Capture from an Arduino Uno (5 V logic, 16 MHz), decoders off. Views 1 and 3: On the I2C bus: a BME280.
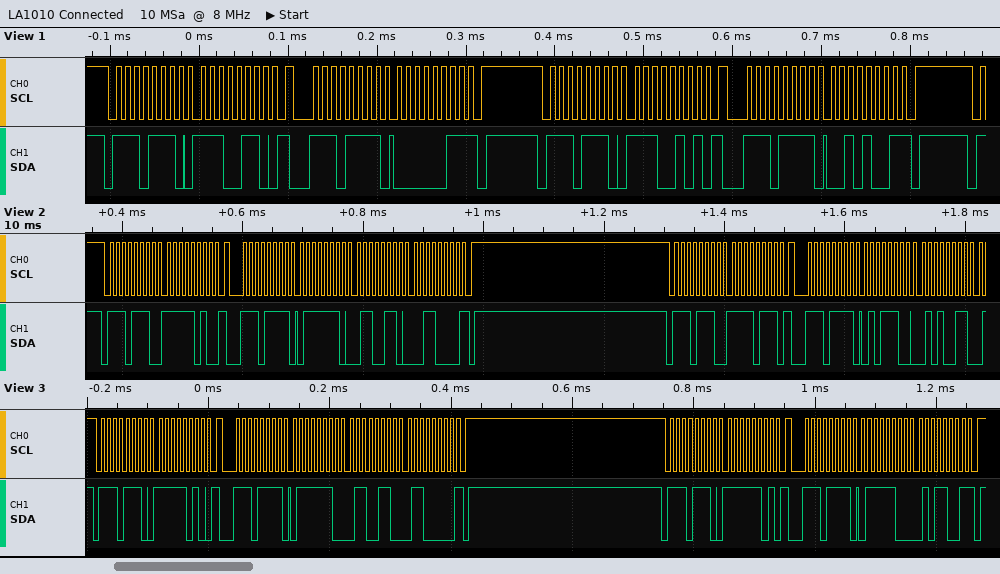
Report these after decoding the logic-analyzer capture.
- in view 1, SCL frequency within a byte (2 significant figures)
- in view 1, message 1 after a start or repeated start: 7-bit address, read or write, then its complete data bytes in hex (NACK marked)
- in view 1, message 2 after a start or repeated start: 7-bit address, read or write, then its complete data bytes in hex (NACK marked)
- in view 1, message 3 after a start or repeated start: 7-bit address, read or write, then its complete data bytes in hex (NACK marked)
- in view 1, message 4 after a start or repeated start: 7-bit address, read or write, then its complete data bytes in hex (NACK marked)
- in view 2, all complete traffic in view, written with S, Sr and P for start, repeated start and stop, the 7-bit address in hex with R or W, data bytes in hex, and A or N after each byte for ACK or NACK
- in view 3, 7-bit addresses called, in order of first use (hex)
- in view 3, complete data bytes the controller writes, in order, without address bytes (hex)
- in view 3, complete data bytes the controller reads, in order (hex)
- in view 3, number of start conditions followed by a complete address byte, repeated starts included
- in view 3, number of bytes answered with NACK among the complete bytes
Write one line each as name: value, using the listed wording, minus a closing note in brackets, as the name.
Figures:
in view 1, SCL frequency within a byte: 100 kHz
in view 1, message 1 after a start or repeated start: 7-bit address, read or write, then its complete data bytes in hex: 0x77 write: E6
in view 1, message 2 after a start or repeated start: 7-bit address, read or write, then its complete data bytes in hex: 0x77 read: 03 NACK
in view 1, message 3 after a start or repeated start: 7-bit address, read or write, then its complete data bytes in hex: 0x77 write: E5
in view 1, message 4 after a start or repeated start: 7-bit address, read or write, then its complete data bytes in hex: 0x77 read: 29 NACK
in view 2, all complete traffic in view, written with S, Sr and P for start, repeated start and stop, the 7-bit address in hex with R or W, data bytes in hex, and A or N after each byte for ACK or NACK: S 77W A FA A Sr 77R A 7E A 66 A 30 N P S 77W A F7 A Sr 77R A 5C A 53 A
in view 3, 7-bit addresses called, in order of first use: 0x77
in view 3, complete data bytes the controller writes, in order, without address bytes: FA FD
in view 3, complete data bytes the controller reads, in order: 7E 66 60 7C 59
in view 3, number of start conditions followed by a complete address byte, repeated starts included: 4
in view 3, number of bytes answered with NACK among the complete bytes: 2
